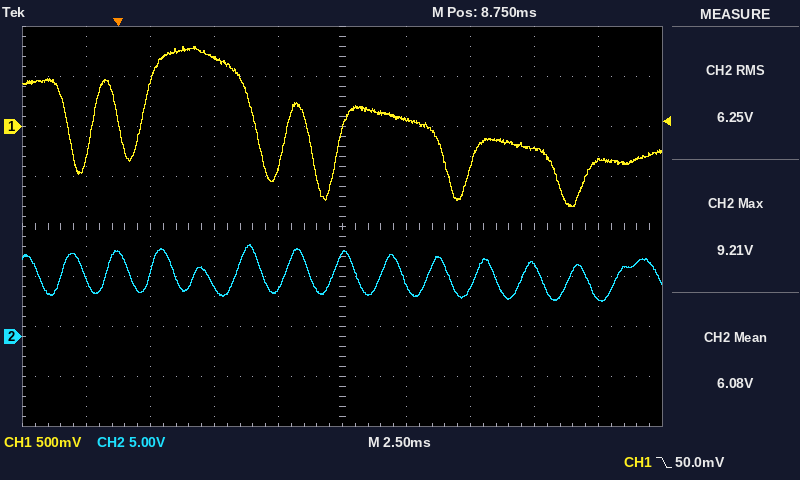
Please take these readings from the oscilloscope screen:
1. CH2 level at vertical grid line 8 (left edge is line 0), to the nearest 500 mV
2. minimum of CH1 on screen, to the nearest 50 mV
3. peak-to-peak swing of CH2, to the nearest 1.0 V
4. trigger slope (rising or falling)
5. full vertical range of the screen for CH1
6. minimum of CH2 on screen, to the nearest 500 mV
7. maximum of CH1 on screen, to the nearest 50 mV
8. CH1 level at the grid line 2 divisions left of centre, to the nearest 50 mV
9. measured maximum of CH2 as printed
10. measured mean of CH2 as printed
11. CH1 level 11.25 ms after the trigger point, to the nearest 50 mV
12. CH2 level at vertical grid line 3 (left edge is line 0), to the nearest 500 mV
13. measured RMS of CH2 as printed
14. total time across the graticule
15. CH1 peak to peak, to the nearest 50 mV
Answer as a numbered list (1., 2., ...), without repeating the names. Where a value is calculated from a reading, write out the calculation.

1. 7.0 V
2. -800 mV
3. 6.0 V
4. falling
5. 4 V
6. 3.5 V
7. 800 mV
8. 700 mV
9. 9.21 V
10. 6.08 V
11. 50 mV
12. 5.0 V
13. 6.25 V
14. 25 ms
15. 800 mV − (-800 mV) = 1.60 V
